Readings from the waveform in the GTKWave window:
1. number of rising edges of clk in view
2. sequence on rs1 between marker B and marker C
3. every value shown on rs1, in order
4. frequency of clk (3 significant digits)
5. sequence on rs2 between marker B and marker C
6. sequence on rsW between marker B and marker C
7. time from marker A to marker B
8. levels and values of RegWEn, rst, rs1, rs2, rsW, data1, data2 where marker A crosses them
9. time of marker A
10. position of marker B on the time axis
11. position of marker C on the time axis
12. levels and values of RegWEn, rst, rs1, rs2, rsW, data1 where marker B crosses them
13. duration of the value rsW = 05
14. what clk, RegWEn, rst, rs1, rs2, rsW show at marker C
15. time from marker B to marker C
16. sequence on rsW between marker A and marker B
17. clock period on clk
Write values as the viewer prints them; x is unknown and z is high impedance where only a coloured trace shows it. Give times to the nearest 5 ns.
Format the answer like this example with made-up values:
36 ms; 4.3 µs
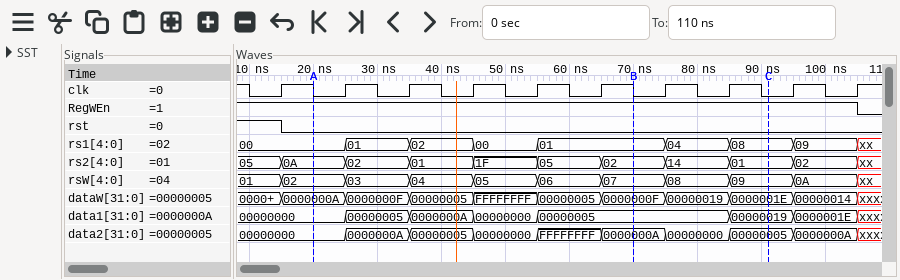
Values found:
10; 01, 04, 08; 00, 01, 02, 00, 01, 04, 08, 09, xx; 100 MHz; 02, 14, 01; 07, 08, 09; 50 ns; RegWEn=1, rst=0, rs1=00, rs2=0A, rsW=02, data1=00000000, data2=00000000; 20 ns; 70 ns; 90 ns; RegWEn=1, rst=0, rs1=01, rs2=02, rsW=07, data1=00000005; 10 ns; clk=0, RegWEn=1, rst=0, rs1=08, rs2=01, rsW=09; 20 ns; 02, 03, 04, 05, 06, 07; 10 ns
